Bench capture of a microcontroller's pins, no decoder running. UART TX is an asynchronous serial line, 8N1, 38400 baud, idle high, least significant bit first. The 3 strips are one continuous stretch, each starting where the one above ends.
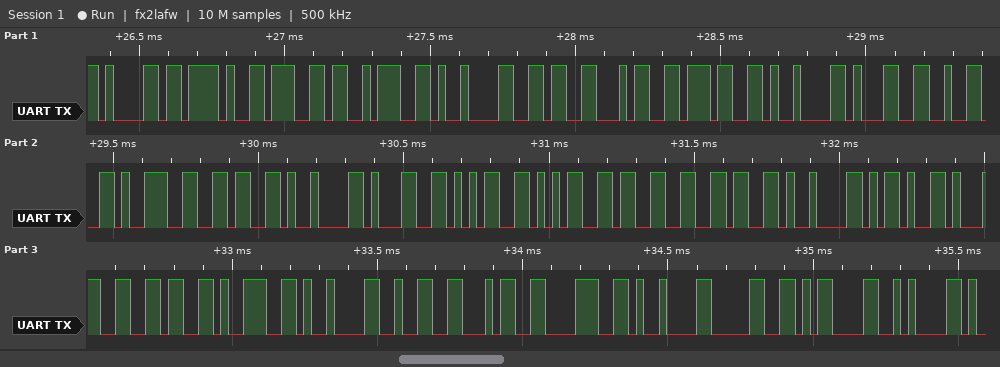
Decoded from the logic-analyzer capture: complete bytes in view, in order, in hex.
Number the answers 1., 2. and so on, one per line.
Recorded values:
1. 61 2F 67 3A 09 36 34 37 09 31 32 39 36 09 31 35 35 33 36 09 2D 31 36 39 09 32 34 38 09 30 0D 0A
